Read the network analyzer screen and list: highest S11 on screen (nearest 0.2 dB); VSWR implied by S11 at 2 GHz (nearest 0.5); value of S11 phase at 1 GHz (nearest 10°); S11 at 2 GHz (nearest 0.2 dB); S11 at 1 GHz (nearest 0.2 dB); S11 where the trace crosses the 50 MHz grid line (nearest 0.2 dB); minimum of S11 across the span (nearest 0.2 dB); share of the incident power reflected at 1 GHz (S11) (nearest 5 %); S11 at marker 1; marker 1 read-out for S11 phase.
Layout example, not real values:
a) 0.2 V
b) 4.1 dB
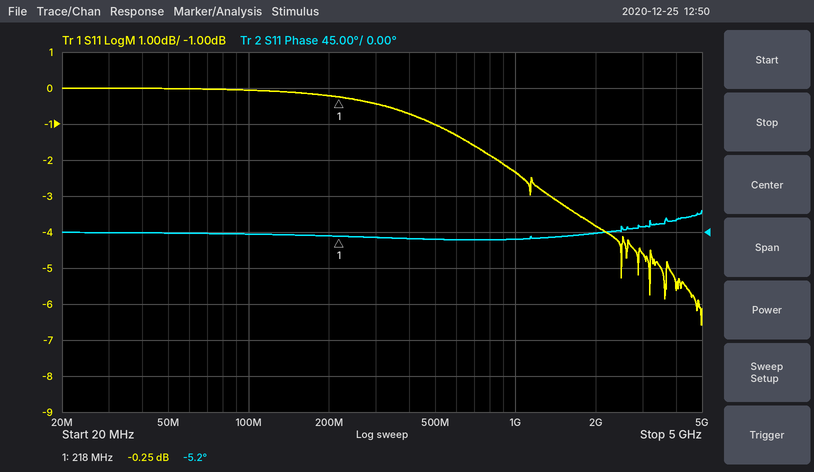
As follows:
a) 0.0 dB
b) 4.5
c) -10°
d) -3.8 dB
e) -2.4 dB
f) 0.0 dB
g) -6.6 dB
h) 60 %
i) -0.25 dB
j) -5.2°
